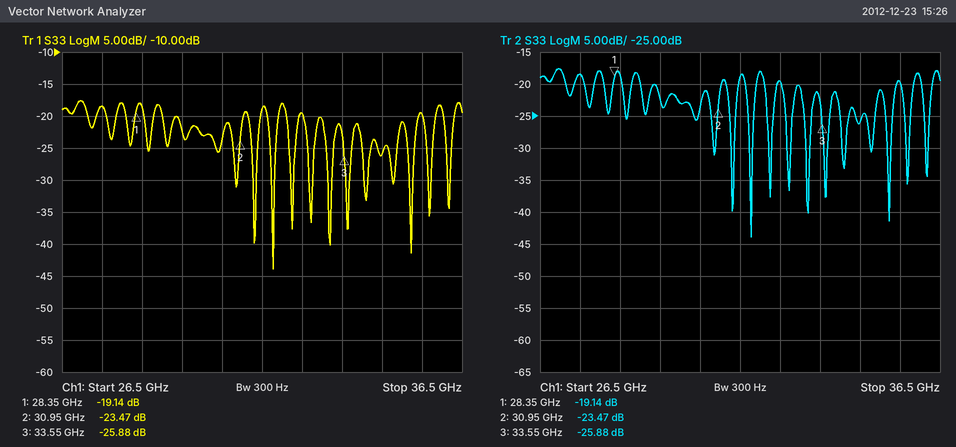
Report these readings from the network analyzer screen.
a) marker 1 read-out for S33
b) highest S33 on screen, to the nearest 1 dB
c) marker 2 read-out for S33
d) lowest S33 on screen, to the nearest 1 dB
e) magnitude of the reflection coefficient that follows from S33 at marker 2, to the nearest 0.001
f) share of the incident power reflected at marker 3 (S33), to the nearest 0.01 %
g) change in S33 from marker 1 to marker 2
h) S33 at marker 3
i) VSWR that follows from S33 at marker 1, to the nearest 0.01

-19.14 dB
-18 dB
-23.47 dB
-44 dB
0.067
0.26 %
-4.33 dB
-25.88 dB
1.25
